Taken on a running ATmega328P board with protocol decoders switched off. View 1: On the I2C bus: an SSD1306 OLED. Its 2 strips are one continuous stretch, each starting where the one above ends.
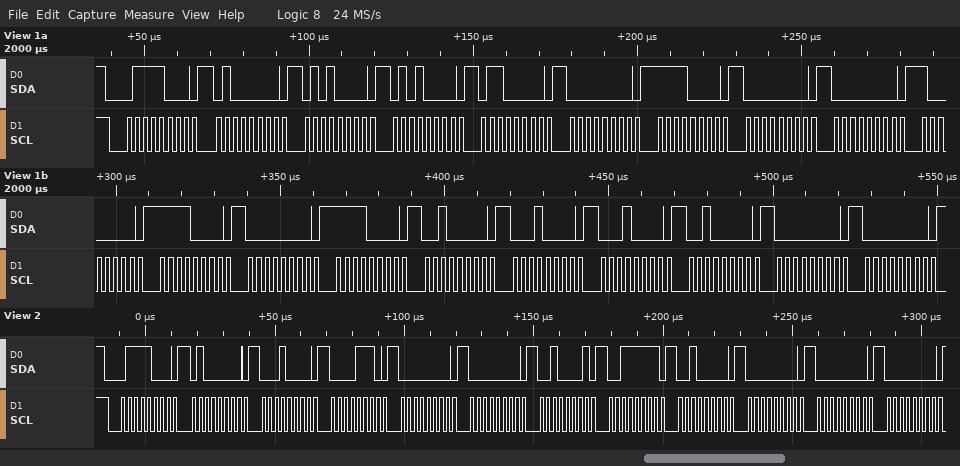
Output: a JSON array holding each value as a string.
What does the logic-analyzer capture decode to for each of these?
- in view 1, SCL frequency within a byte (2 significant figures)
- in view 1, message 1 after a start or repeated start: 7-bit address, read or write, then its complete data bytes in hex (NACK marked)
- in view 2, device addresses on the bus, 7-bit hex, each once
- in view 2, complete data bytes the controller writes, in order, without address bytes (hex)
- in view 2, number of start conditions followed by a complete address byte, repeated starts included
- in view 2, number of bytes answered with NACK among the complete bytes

["400 kHz", "0x3C write: 40 50 50 60 00 F0 00 00 80 F0 00 F0 20 10 10 20 00 00", "0x3C", "40 10 0E 00 00 21 3F 20 00 00 00", "1", "0"]
